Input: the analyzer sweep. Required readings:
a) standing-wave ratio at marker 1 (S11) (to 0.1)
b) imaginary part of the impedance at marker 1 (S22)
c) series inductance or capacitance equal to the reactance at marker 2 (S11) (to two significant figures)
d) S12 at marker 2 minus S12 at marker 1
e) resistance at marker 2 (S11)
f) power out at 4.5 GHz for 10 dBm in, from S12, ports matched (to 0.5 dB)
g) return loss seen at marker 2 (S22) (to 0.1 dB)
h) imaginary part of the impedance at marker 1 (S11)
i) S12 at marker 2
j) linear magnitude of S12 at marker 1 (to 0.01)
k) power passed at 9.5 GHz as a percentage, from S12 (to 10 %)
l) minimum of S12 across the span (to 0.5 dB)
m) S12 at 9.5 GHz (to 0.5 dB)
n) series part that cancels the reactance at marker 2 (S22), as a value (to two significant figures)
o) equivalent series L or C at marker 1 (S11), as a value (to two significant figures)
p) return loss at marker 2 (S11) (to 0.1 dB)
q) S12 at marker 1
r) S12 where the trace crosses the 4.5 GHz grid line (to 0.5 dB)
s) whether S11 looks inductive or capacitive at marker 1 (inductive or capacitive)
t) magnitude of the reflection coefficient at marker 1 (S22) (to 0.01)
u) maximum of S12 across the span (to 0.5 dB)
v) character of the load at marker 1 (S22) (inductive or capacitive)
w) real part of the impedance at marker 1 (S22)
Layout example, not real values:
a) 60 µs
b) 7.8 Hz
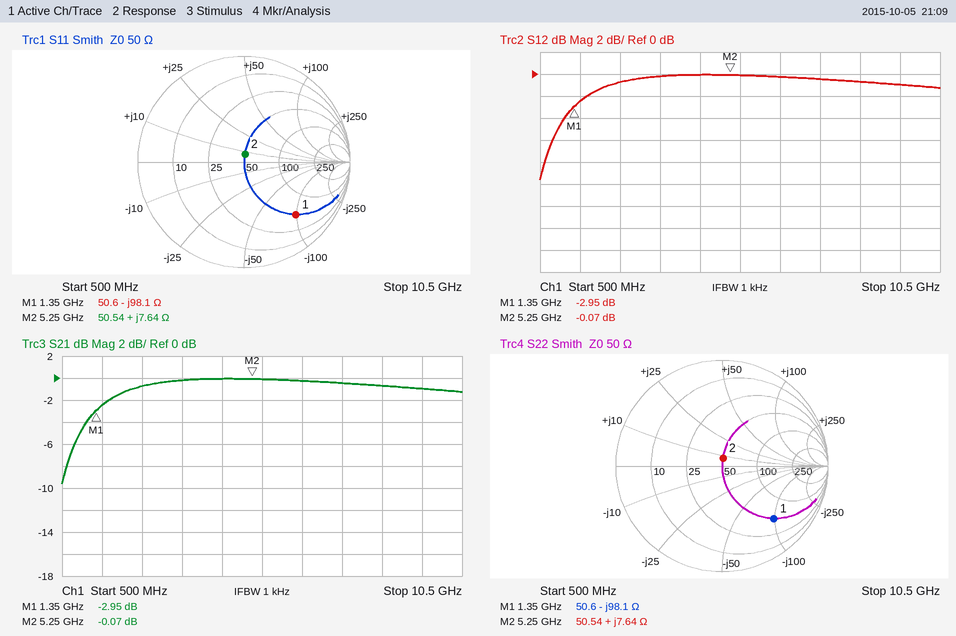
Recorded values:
a) 5.6
b) -98.1 Ω
c) 230 pH
d) 2.88 dB
e) 50.54 Ω
f) 10.0 dBm
g) 22.4 dB
h) -98.1 Ω
i) -0.07 dB
j) 0.71
k) 80 %
l) -9.5 dB
m) -1.0 dB
n) 4.0 pF
o) 1.2 pF
p) 22.4 dB
q) -2.95 dB
r) 0.0 dB
s) capacitive
t) 0.70
u) 0.0 dB
v) capacitive
w) 50.6 Ω
